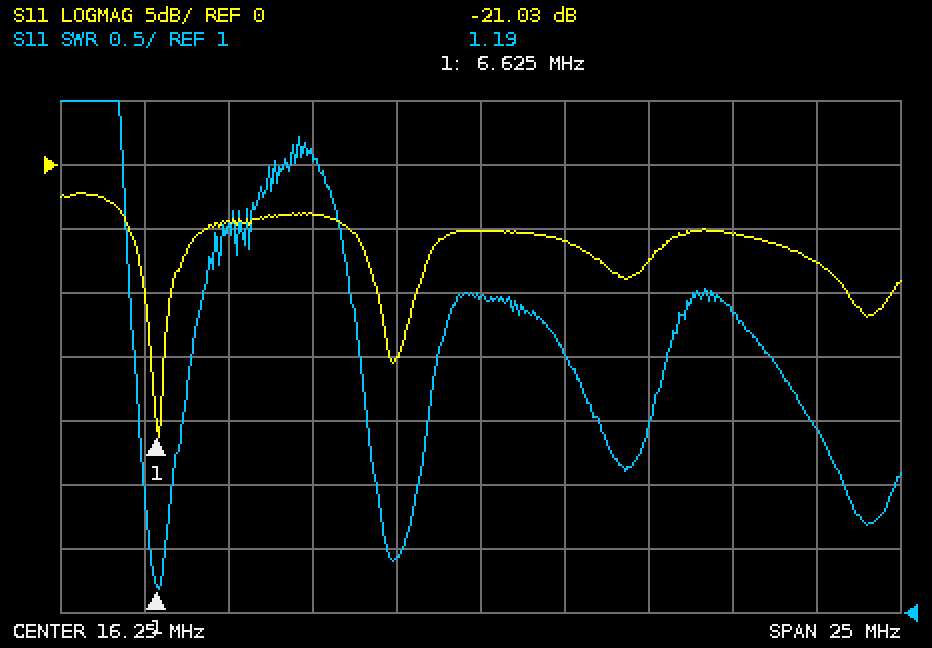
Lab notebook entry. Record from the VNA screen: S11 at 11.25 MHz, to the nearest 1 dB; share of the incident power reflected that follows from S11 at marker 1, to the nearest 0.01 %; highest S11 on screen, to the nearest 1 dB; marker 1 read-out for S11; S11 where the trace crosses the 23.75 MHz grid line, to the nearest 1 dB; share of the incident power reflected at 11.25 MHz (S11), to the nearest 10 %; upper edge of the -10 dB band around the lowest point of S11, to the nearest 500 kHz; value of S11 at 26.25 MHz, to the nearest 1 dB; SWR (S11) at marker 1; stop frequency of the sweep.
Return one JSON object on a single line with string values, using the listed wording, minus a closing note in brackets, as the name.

{"S11 at 11.25 MHz, to the nearest 1 dB": "-4 dB", "share of the incident power reflected that follows from S11 at marker 1, to the nearest 0.01 %": "0.79 %", "highest S11 on screen, to the nearest 1 dB": "-2 dB", "marker 1 read-out for S11": "-21.03 dB", "S11 where the trace crosses the 23.75 MHz grid line, to the nearest 1 dB": "-5 dB", "share of the incident power reflected at 11.25 MHz (S11), to the nearest 10 %": "40 %", "upper edge of the -10 dB band around the lowest point of S11, to the nearest 500 kHz": "7.0 MHz", "value of S11 at 26.25 MHz, to the nearest 1 dB": "-8 dB", "SWR (S11) at marker 1": "1.19", "stop frequency of the sweep": "28.75 MHz"}
